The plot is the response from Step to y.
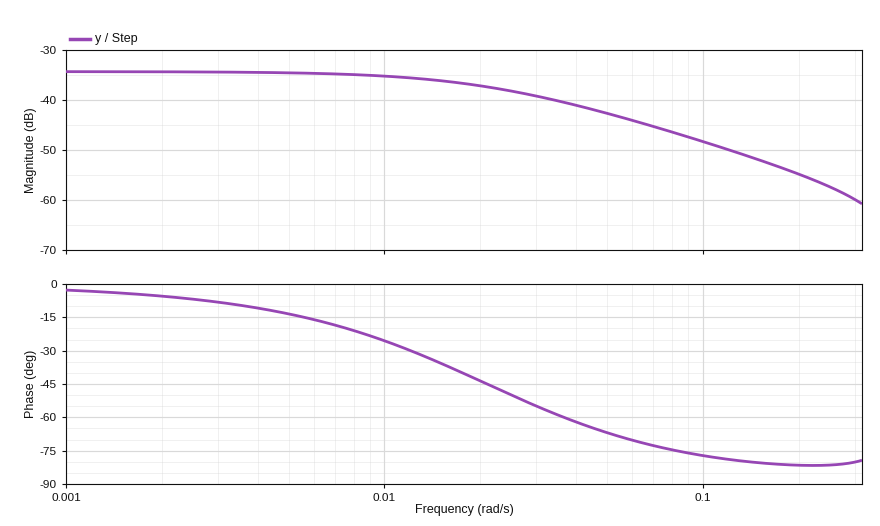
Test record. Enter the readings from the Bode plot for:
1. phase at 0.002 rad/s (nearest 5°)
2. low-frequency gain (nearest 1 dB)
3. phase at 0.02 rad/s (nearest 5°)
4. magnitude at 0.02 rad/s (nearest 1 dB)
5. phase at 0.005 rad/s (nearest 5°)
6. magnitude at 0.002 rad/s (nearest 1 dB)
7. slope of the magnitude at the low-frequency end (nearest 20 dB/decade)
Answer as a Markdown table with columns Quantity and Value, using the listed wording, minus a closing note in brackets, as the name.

| Quantity | Value |
|---|---|
| phase at 0.002 rad/s | -5° |
| low-frequency gain | -34 dB |
| phase at 0.02 rad/s | -45° |
| magnitude at 0.02 rad/s | -37 dB |
| phase at 0.005 rad/s | -15° |
| magnitude at 0.002 rad/s | -34 dB |
| slope of the magnitude at the low-frequency end | 0 dB/decade |
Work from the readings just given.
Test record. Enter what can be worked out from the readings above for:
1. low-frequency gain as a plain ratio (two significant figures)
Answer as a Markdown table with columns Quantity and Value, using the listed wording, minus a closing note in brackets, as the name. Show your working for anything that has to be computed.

| Quantity | Value |
|---|---|
| low-frequency gain as a plain ratio | 10^(-34 / 20) = 0.020 |
